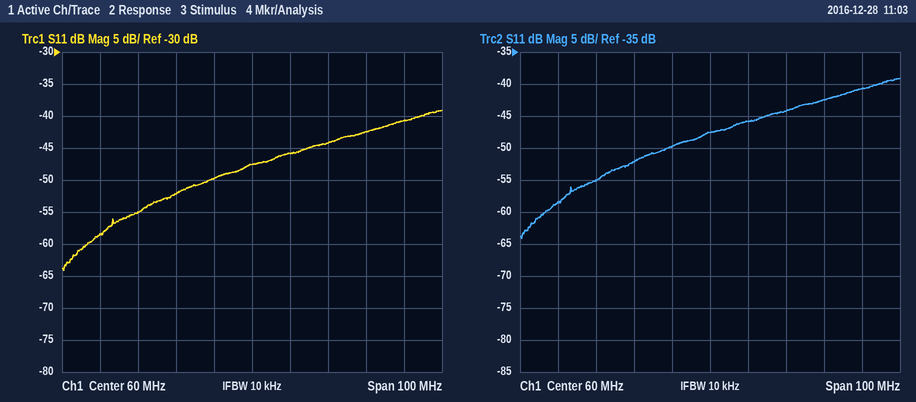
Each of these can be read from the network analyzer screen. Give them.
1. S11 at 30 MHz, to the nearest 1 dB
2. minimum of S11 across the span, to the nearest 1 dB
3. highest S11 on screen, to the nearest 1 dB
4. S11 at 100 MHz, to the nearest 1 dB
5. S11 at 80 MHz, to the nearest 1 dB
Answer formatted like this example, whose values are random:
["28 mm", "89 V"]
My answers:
["-55 dB", "-64 dB", "-39 dB", "-41 dB", "-44 dB"]
